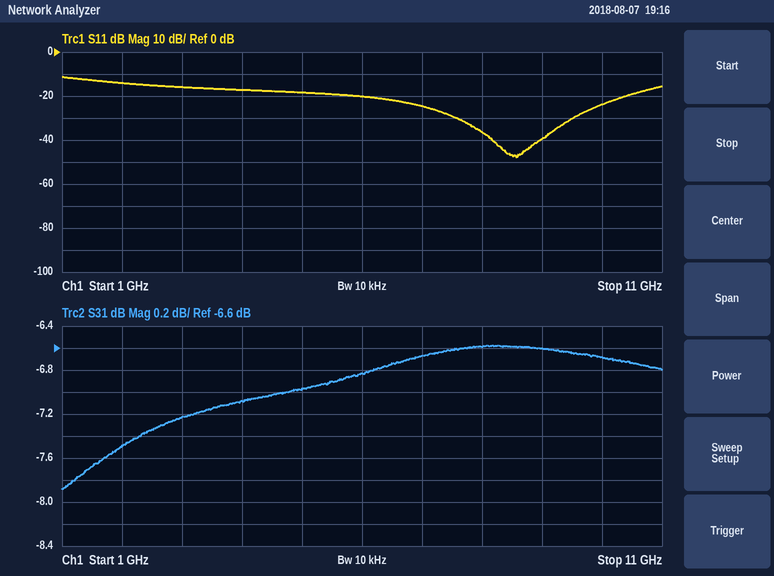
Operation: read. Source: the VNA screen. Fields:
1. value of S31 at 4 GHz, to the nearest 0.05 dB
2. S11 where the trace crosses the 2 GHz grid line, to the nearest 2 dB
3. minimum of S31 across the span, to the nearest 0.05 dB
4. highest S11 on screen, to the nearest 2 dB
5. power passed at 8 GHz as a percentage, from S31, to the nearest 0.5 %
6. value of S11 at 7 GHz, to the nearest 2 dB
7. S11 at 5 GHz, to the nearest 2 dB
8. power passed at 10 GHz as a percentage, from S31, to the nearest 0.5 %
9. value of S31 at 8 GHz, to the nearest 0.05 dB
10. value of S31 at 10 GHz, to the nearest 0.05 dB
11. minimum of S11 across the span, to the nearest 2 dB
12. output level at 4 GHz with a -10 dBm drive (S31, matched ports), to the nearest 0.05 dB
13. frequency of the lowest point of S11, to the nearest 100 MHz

-7.10 dB
-14 dB
-7.90 dB
-12 dB
22.0 %
-24 dB
-18 dB
21.5 %
-6.60 dB
-6.70 dB
-48 dB
-17.10 dBm
8.6 GHz
